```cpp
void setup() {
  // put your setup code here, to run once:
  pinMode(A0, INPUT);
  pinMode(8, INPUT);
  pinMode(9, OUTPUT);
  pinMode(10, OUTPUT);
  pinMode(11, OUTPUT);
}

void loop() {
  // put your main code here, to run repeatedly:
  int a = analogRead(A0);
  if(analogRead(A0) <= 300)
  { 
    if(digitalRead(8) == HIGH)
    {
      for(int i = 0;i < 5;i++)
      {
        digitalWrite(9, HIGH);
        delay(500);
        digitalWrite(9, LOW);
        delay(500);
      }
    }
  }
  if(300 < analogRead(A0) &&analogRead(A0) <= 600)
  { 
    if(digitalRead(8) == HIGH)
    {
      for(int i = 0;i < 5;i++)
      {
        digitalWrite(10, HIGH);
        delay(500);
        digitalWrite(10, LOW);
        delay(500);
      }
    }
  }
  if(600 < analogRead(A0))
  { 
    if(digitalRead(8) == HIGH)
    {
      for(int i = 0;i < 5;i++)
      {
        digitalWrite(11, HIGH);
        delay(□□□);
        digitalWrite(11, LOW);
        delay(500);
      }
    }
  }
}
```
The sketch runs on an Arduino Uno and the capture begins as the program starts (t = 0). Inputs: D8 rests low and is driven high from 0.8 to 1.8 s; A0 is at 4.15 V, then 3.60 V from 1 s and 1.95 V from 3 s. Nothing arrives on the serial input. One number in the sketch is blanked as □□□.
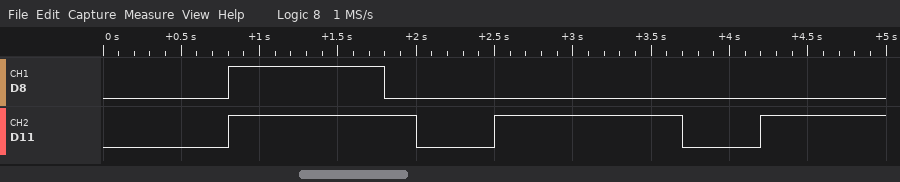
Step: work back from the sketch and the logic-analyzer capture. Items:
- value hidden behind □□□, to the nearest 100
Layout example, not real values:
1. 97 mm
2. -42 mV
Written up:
1. 1200
